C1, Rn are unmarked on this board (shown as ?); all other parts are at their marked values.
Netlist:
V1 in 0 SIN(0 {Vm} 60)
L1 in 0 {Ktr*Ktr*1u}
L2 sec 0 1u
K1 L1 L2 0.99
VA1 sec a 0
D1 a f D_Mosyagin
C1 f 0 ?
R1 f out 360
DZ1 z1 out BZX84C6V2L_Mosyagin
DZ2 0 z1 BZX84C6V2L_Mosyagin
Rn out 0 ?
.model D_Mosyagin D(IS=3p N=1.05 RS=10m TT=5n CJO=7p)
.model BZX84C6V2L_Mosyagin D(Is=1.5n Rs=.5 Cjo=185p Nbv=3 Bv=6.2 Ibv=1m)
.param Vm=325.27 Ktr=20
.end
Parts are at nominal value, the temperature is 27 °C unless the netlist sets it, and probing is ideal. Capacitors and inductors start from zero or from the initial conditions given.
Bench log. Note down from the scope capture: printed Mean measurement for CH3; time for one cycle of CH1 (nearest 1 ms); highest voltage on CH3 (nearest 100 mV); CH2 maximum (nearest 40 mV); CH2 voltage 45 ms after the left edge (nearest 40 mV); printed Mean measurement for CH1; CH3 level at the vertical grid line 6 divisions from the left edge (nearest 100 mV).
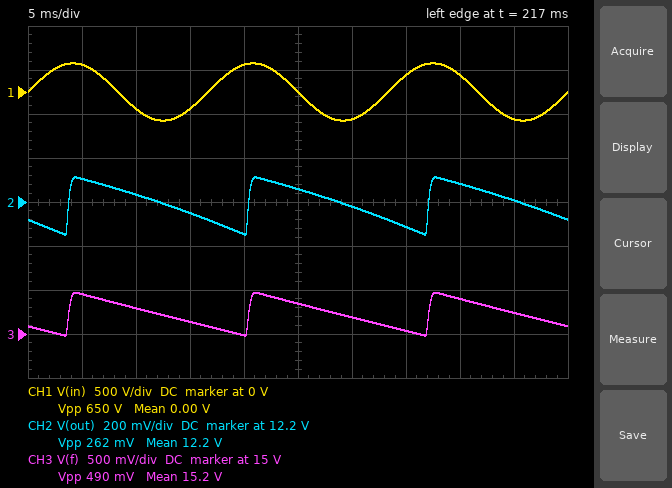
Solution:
15.2 V
17 ms
15.5 V
12.32 V
12.20 V
0.00 V
15.2 V
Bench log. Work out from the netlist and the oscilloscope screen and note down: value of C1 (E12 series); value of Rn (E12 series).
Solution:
270 µF
1.5 kΩ
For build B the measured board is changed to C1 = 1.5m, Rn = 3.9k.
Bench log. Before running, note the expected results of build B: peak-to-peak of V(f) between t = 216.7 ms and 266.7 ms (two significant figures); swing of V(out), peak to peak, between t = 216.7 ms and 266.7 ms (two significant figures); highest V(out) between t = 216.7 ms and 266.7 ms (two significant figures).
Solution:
81 mV
7.4 mV
13 V
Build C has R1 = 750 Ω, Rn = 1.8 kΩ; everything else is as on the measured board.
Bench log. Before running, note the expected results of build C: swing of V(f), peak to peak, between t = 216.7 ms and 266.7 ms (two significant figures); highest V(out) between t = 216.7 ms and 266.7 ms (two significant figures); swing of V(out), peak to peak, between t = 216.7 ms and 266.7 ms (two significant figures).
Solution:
350 mV
11 V
250 mV
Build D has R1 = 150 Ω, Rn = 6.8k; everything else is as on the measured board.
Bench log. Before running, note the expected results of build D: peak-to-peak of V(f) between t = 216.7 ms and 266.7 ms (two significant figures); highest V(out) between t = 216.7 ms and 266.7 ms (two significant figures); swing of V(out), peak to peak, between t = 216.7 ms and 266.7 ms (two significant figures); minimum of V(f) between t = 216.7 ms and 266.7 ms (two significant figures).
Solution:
850 mV
13 V
68 mV
15 V
